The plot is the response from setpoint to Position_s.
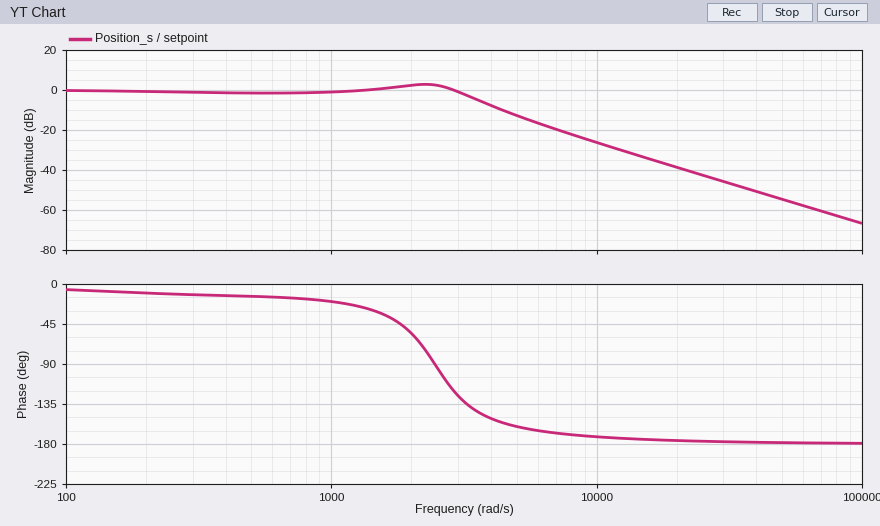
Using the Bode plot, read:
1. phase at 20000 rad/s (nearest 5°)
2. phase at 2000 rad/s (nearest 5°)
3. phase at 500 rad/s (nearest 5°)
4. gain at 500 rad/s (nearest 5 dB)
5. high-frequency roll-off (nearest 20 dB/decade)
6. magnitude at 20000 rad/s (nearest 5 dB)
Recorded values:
-175°
-55°
-15°
0 dB
-40 dB/decade
-40 dB
